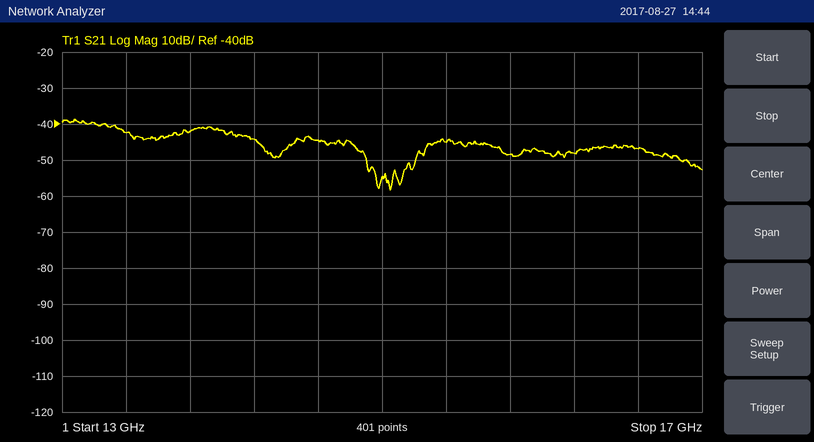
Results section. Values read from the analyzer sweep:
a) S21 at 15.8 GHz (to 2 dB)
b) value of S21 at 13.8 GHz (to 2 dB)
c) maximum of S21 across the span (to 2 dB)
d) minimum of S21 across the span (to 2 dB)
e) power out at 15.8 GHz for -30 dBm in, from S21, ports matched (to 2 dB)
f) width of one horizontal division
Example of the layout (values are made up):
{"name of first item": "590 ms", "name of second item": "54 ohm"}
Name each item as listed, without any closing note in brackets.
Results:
{"S21 at 15.8 GHz": "-48 dB", "value of S21 at 13.8 GHz": "-42 dB", "maximum of S21 across the span": "-38 dB", "minimum of S21 across the span": "-58 dB", "power out at 15.8 GHz for -30 dBm in, from S21, ports matched": "-78 dBm", "width of one horizontal division": "400 MHz"}
